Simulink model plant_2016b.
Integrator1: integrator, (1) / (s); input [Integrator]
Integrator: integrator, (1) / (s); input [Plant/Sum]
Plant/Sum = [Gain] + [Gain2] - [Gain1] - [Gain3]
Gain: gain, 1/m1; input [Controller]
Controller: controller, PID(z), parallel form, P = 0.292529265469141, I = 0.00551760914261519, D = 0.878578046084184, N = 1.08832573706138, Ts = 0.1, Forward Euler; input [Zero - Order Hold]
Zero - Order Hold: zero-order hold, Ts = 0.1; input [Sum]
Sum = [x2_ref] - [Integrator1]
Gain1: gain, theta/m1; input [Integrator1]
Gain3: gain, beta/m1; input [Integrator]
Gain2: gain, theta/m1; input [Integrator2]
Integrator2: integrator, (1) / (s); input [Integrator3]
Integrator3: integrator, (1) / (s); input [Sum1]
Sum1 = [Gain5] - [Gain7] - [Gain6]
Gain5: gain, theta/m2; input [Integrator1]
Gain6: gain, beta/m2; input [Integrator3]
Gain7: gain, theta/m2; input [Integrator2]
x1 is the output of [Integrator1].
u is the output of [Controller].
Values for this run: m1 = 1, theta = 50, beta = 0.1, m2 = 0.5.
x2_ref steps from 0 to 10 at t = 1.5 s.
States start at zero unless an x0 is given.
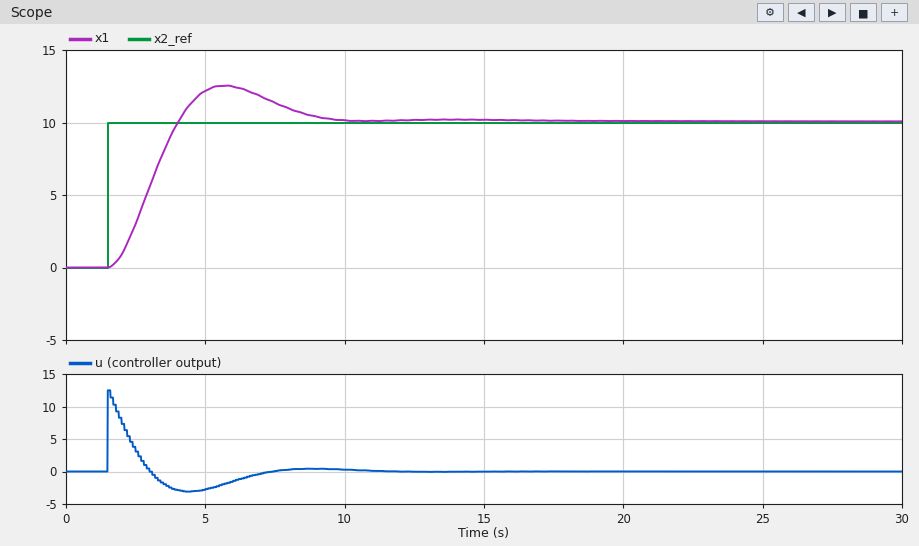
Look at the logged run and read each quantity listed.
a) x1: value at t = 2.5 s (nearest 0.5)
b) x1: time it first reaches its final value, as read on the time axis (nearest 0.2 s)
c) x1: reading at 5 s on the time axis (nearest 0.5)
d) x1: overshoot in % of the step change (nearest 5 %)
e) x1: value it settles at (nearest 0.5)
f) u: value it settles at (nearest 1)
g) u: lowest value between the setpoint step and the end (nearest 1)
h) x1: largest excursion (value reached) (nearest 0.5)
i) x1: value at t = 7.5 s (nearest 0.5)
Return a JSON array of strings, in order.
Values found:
["3.0", "4.0 s", "12.0", "25 %", "10.0", "0", "-3", "12.5", "11.5"]
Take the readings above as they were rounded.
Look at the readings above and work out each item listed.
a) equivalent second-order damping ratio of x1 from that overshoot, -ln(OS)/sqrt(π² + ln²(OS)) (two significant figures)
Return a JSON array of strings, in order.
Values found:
["0.40"]
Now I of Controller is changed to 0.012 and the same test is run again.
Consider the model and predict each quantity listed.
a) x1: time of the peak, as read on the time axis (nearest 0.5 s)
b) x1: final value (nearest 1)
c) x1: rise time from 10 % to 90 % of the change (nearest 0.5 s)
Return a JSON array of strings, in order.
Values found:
["6.0 s", "10", "1.5 s"]
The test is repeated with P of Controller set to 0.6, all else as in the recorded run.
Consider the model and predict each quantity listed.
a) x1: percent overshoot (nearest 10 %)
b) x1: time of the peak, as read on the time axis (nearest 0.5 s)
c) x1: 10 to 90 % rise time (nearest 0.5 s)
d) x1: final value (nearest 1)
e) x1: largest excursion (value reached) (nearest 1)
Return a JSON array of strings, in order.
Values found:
["40 %", "5.0 s", "1.5 s", "10", "14"]
